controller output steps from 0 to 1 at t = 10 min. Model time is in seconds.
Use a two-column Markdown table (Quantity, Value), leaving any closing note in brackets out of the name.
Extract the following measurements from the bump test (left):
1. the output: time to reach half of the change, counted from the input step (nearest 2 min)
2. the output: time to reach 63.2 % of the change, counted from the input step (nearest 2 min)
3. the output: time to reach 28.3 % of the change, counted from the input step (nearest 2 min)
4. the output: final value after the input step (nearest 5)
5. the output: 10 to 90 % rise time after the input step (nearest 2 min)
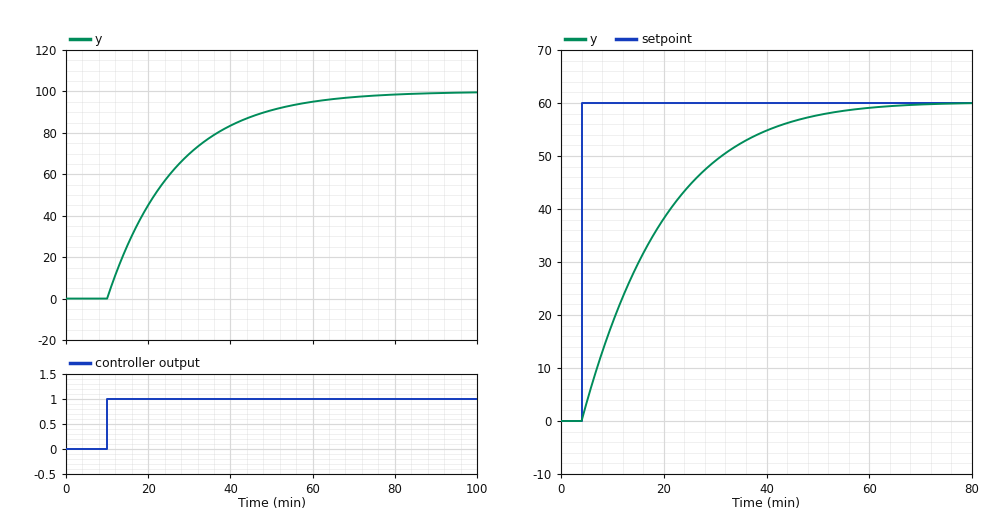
| Quantity | Value |
|---|---|
| the output: time to reach half of the change, counted from the input step | 12 min |
| the output: time to reach 63.2 % of the change, counted from the input step | 16 min |
| the output: time to reach 28.3 % of the change, counted from the input step | 6 min |
| the output: final value after the input step | 100 |
| the output: 10 to 90 % rise time after the input step | 36 min |
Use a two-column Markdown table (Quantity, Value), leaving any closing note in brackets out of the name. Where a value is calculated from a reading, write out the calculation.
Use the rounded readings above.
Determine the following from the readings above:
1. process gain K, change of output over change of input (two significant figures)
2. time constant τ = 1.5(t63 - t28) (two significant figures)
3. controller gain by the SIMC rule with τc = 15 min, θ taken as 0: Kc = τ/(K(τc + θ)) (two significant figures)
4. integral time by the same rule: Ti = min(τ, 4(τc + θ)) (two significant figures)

| Quantity | Value |
|---|---|
| process gain K, change of output over change of input | (100 - 0) / 1 = 100 |
| time constant τ = 1.5(t63 - t28) | 1.5 × (16 - 6) = 15 min |
| controller gain by the SIMC rule with τc = 15 min, θ taken as 0: Kc = τ/(K(τc + θ)) | 15 / (100 × (15 + 0)) = 0.010 |
| integral time by the same rule: Ti = min(τ, 4(τc + θ)) | min(15, 4 × (15 + 0)) = 15 min |
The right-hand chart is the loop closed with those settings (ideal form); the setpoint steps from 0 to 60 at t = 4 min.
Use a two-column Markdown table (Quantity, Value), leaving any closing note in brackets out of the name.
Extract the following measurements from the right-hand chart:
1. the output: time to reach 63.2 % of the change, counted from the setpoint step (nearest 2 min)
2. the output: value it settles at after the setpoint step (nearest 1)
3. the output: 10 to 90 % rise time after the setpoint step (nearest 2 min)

| Quantity | Value |
|---|---|
| the output: time to reach 63.2 % of the change, counted from the setpoint step | 16 min |
| the output: value it settles at after the setpoint step | 60 |
| the output: 10 to 90 % rise time after the setpoint step | 32 min |
